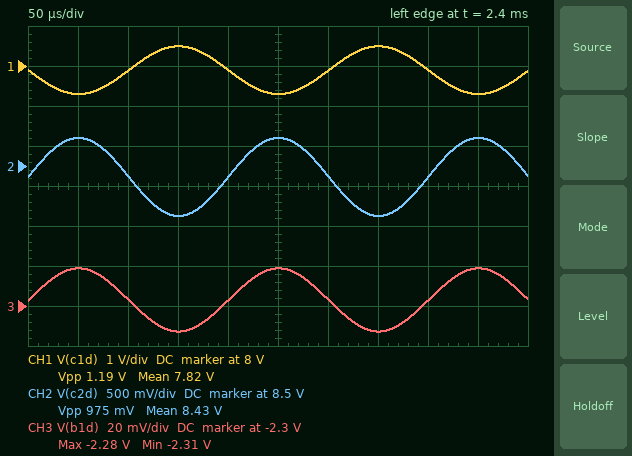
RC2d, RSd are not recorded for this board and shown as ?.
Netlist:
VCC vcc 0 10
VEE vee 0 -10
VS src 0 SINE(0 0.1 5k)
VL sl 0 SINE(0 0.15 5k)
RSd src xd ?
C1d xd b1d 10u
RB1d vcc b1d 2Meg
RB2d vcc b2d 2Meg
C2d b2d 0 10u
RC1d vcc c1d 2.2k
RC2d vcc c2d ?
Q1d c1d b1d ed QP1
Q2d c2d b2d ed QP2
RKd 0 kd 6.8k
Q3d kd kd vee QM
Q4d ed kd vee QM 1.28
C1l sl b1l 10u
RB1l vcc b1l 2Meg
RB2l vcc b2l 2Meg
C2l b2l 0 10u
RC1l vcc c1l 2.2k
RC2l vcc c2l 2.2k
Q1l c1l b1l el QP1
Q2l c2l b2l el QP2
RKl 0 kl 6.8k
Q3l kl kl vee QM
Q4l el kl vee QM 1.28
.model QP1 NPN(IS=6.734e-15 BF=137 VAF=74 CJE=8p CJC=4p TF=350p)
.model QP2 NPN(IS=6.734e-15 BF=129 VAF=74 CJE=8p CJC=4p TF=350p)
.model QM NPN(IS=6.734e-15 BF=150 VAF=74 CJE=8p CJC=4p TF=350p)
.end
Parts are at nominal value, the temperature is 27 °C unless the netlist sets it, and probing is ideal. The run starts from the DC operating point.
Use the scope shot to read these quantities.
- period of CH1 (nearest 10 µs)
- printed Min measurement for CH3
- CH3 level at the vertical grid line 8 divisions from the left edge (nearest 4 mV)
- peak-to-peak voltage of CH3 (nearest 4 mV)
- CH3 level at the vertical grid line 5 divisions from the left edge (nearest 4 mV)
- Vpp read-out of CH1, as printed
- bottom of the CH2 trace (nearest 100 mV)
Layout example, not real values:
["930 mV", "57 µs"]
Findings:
["200 µs", "-2.31 V", "-2.296 V", "32 mV", "-2.280 V", "1.19 V", "7.9 V"]
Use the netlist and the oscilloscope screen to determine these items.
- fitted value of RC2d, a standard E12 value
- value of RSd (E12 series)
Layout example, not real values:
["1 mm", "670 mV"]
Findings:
["1.8 kΩ", "47 kΩ"]
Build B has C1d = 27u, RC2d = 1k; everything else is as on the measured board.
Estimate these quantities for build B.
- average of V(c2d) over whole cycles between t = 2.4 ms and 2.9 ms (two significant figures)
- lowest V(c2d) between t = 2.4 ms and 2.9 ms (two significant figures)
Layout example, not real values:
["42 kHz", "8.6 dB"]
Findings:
["9.1 V", "8.8 V"]
